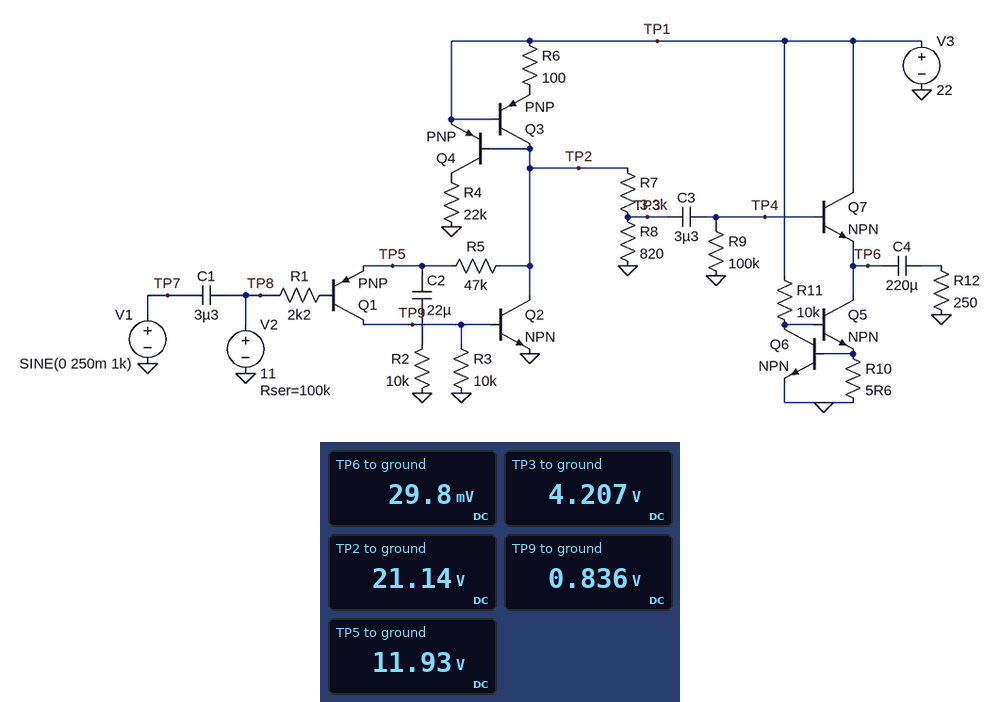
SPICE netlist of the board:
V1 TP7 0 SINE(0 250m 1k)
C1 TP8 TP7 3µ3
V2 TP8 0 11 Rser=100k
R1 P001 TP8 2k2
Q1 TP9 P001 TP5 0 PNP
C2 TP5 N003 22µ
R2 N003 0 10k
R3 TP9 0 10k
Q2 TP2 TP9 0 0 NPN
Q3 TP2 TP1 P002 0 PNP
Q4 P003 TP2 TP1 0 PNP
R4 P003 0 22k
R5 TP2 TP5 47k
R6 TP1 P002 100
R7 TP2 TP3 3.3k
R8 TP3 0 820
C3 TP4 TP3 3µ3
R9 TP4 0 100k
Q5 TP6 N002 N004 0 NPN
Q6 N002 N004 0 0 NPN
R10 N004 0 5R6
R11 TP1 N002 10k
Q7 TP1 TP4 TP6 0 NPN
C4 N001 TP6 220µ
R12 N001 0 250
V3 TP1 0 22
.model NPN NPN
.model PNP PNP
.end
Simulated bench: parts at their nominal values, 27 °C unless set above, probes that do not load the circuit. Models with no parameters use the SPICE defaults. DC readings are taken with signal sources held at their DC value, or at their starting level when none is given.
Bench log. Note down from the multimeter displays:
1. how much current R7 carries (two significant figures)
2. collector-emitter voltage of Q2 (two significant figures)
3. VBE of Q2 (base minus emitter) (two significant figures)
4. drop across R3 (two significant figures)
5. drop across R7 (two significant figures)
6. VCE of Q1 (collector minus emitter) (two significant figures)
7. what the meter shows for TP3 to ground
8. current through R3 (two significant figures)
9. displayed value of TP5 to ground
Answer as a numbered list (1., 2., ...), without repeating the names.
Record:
1. 5.1 mA
2. 21 V
3. 840 mV
4. 840 mV
5. 17 V
6. -11 V
7. 4.207 V
8. 84 µA
9. 11.93 V
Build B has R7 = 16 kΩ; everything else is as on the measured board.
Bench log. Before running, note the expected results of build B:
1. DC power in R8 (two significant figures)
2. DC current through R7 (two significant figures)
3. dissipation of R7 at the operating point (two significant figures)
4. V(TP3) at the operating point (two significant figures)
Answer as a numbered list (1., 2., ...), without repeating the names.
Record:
1. 1.3 mW
2. 1.3 mA
3. 25 mW
4. 1.0 V
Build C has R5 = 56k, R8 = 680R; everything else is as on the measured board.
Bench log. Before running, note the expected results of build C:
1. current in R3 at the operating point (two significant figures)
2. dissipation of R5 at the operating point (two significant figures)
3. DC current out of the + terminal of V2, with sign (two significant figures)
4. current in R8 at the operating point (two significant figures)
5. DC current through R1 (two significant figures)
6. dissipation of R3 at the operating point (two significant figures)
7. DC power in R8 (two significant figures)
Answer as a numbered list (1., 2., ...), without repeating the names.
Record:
1. 83 µA
2. 1.5 mW
3. -1.6 µA
4. 5.3 mA
5. 1.6 µA
6. 69 µW
7. 19 mW
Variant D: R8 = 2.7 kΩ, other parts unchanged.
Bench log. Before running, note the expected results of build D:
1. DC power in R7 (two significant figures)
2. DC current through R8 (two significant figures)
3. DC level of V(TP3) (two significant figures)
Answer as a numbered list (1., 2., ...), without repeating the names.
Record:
1. 41 mW
2. 3.5 mA
3. 9.5 V
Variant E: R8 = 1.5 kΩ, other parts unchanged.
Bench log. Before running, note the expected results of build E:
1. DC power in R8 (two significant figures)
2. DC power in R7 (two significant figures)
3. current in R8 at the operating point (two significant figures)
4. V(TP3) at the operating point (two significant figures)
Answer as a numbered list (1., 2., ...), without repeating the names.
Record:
1. 29 mW
2. 64 mW
3. 4.4 mA
4. 6.6 V
